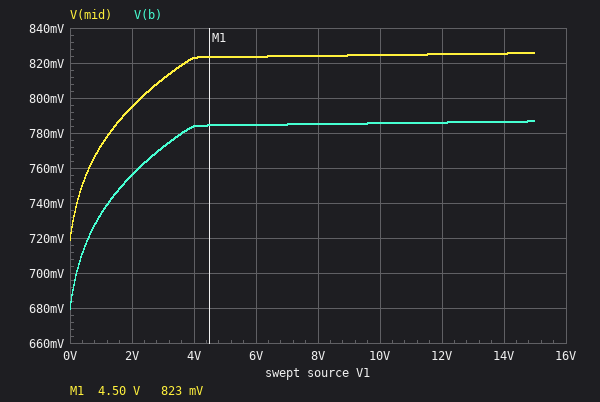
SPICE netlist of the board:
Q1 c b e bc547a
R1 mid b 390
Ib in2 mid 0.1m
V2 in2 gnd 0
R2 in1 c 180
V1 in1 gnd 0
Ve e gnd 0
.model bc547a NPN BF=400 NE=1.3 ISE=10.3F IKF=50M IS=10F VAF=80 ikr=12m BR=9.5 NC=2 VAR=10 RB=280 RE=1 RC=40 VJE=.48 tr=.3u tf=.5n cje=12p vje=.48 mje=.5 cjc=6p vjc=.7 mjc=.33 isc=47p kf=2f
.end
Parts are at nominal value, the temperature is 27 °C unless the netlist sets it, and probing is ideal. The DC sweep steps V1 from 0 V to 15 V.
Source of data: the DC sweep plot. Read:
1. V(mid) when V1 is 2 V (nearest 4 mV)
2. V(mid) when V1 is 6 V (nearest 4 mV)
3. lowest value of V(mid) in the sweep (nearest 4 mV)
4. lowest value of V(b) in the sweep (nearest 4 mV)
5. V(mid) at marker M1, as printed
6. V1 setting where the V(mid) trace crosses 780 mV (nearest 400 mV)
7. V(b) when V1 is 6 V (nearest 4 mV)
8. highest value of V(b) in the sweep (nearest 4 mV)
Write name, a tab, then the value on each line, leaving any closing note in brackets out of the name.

V(mid) when V1 is 2 V	796 mV
V(mid) when V1 is 6 V	824 mV
lowest value of V(mid) in the sweep	720 mV
lowest value of V(b) in the sweep	680 mV
V(mid) at marker M1, as printed	823 mV
V1 setting where the V(mid) trace crosses 780 mV	1.2 V
V(b) when V1 is 6 V	784 mV
highest value of V(b) in the sweep	788 mV
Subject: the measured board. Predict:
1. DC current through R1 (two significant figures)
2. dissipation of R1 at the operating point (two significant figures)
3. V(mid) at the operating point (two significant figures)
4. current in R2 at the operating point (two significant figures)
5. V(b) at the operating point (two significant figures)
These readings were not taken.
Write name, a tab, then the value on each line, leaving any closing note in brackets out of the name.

DC current through R1	100 µA
dissipation of R1 at the operating point	3.9 µW
V(mid) at the operating point	720 mV
current in R2 at the operating point	14 µA
V(b) at the operating point	680 mV
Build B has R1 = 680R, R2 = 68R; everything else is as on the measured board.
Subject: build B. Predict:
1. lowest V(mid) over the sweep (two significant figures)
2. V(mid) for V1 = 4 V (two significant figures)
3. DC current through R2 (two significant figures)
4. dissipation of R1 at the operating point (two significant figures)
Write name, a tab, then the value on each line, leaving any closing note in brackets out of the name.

lowest V(mid) over the sweep	750 mV
V(mid) for V1 = 4 V	850 mV
DC current through R2	25 µA
dissipation of R1 at the operating point	6.8 µW
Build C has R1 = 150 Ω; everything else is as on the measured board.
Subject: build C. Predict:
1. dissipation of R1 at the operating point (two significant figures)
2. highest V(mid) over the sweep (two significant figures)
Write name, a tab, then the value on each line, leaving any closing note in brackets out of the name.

dissipation of R1 at the operating point	1.5 µW
highest V(mid) over the sweep	800 mV
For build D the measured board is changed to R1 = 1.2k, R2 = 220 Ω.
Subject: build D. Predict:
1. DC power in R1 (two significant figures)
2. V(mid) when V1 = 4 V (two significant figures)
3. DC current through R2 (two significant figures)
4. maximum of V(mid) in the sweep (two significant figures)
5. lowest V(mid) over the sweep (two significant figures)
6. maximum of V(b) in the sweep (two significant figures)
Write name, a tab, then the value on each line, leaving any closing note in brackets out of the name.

DC power in R1	12 µW
V(mid) when V1 = 4 V	900 mV
DC current through R2	12 µA
maximum of V(mid) in the sweep	910 mV
lowest V(mid) over the sweep	800 mV
maximum of V(b) in the sweep	790 mV
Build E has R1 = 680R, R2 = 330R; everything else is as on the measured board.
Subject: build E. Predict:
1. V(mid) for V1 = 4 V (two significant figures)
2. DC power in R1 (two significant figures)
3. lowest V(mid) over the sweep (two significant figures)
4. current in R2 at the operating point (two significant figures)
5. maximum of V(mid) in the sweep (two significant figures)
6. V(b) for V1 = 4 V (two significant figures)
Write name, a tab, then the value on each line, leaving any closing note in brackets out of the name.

V(mid) for V1 = 4 V	830 mV
DC power in R1	6.8 µW
lowest V(mid) over the sweep	750 mV
current in R2 at the operating point	8.7 µA
maximum of V(mid) in the sweep	850 mV
V(b) for V1 = 4 V	760 mV
